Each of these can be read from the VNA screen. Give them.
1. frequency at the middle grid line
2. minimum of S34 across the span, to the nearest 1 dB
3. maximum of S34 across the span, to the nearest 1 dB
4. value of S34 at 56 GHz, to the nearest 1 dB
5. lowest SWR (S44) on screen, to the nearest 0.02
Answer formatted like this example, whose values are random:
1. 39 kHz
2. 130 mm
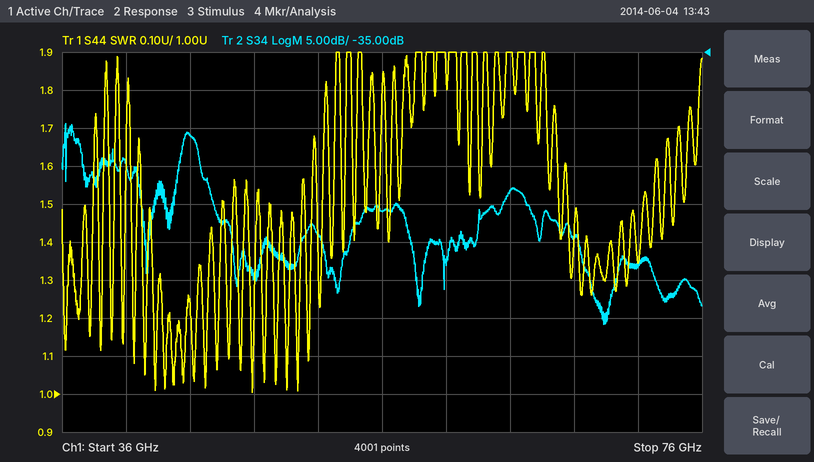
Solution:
1. 56 GHz
2. -71 dB
3. -44 dB
4. -56 dB
5. 1.00
